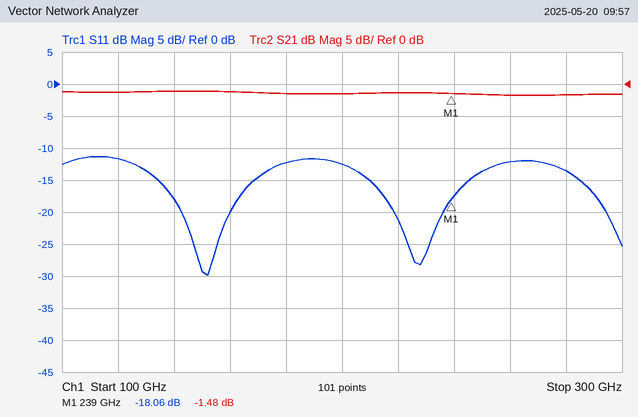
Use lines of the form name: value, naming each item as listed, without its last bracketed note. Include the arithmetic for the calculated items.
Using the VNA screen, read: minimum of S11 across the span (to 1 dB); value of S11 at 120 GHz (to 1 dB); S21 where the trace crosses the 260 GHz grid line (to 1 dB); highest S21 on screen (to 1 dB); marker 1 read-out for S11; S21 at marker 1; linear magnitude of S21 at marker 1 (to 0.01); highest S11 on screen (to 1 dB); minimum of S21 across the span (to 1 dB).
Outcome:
minimum of S11 across the span: -30 dB
value of S11 at 120 GHz: -12 dB
S21 where the trace crosses the 260 GHz grid line: -2 dB
highest S21 on screen: -1 dB
marker 1 read-out for S11: -18.06 dB
S21 at marker 1: -1.48 dB
linear magnitude of S21 at marker 1: 10^(-1.48/20) ≈ 0.84
highest S11 on screen: -11 dB
minimum of S21 across the span: -2 dB
